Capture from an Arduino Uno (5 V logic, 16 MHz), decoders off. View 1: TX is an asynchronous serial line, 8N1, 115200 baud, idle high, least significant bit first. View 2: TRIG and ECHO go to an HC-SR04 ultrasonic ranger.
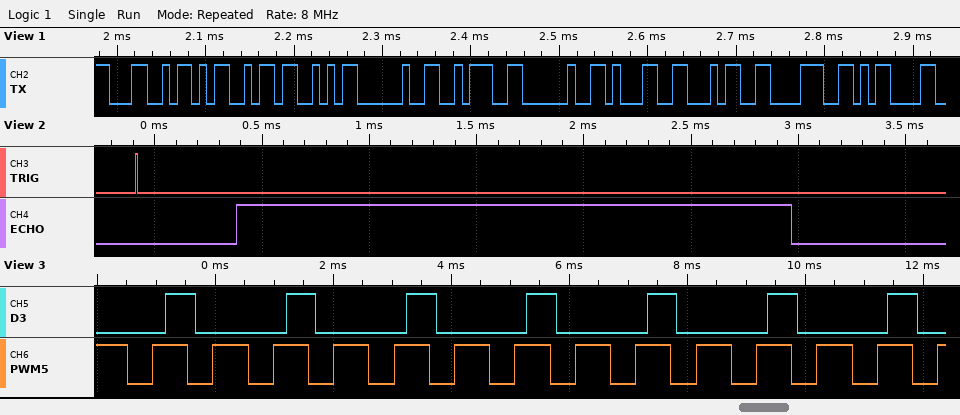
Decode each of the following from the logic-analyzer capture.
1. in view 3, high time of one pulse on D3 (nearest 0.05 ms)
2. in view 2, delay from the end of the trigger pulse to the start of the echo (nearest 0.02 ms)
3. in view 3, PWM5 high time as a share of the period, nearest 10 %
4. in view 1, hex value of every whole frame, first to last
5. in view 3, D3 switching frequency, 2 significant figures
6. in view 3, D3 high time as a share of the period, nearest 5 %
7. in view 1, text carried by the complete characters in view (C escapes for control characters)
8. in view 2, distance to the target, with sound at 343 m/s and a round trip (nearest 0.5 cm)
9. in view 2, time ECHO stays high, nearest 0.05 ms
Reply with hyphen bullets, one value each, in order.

- 0.50 ms
- 0.46 ms
- 60 %
- 4C 4D 53 20 3A 20 31 34 38 0D
- 490 Hz
- 25 %
- "LMS : 148\r"
- 44.5 cm
- 2.60 ms
